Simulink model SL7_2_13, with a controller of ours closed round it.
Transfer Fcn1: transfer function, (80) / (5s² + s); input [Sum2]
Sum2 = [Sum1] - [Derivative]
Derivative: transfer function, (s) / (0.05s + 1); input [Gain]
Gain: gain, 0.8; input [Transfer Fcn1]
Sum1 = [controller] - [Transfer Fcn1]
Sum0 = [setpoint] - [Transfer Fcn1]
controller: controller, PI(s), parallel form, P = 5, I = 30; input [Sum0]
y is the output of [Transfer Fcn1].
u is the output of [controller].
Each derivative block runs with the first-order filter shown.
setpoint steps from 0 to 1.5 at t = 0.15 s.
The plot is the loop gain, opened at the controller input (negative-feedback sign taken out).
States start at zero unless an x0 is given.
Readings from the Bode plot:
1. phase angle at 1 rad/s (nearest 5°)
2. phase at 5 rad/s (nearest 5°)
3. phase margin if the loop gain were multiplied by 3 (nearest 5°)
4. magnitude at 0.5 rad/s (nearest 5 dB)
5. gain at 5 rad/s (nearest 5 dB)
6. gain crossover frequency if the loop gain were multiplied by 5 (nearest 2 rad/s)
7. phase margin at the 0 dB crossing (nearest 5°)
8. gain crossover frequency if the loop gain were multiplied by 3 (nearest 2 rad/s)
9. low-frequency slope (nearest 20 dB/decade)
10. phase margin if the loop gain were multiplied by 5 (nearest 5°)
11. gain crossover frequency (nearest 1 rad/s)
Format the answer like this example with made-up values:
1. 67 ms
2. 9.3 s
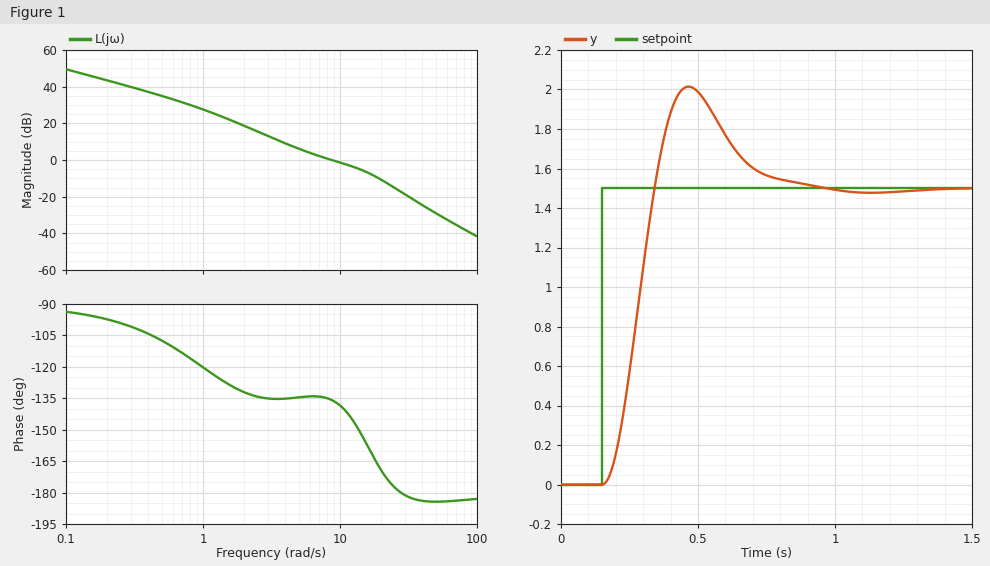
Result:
1. -120°
2. -135°
3. 15°
4. 35 dB
5. 5 dB
6. 24 rad/s
7. 45°
8. 18 rad/s
9. -20 dB/decade
10. 5°
11. 9 rad/s
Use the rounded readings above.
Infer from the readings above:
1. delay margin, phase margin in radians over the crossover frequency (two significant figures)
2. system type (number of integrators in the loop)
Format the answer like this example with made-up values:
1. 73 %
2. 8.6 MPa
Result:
1. 0.087 s
2. 1
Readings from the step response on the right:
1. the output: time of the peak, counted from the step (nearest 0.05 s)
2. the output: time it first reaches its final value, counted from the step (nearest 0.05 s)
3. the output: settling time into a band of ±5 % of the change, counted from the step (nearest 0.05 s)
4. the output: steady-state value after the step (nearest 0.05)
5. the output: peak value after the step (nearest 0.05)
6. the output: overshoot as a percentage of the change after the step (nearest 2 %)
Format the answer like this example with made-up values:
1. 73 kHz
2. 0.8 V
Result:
1. 0.30 s
2. 0.20 s
3. 0.60 s
4. 1.50
5. 2.00
6. 34 %
